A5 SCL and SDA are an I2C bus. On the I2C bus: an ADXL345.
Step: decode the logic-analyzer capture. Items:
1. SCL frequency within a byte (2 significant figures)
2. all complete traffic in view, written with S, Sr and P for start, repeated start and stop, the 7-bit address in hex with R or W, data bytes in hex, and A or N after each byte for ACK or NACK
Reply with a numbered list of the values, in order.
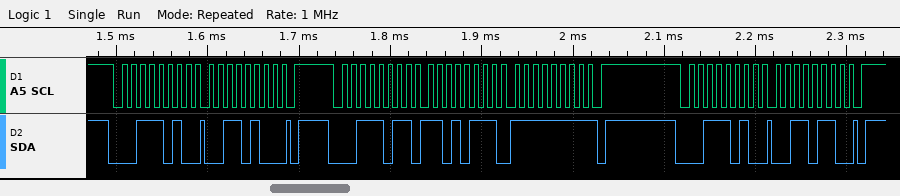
1. 100 kHz
2. S 1DW A 34 A P S 1DR A D7 A FF N P S 1DW A 36 A P
